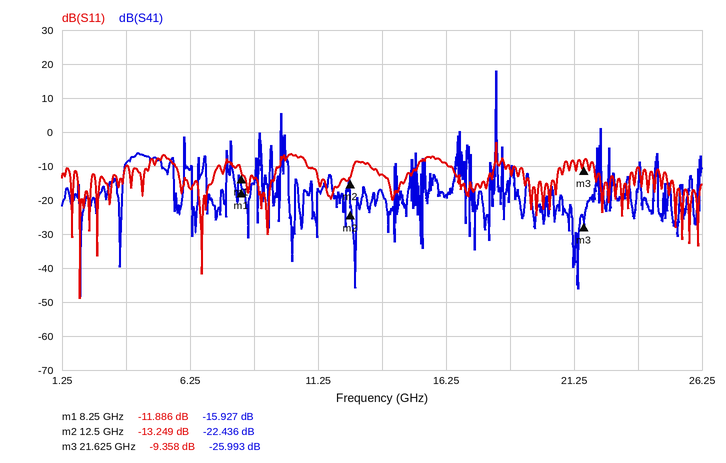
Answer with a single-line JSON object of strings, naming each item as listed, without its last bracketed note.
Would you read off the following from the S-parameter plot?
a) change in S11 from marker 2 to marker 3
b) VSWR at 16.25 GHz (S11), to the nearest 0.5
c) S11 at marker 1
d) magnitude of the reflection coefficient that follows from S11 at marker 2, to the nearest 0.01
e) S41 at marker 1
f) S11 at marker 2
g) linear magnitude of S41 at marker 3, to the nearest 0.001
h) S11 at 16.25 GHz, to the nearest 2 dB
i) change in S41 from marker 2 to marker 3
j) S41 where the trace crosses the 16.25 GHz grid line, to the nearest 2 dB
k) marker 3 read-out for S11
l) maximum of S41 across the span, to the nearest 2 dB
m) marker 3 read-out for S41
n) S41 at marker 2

{"change in S11 from marker 2 to marker 3": "3.891 dB", "VSWR at 16.25 GHz (S11), to the nearest 0.5": "2.0", "S11 at marker 1": "-11.886 dB", "magnitude of the reflection coefficient that follows from S11 at marker 2, to the nearest 0.01": "0.22", "S41 at marker 1": "-15.927 dB", "S11 at marker 2": "-13.249 dB", "linear magnitude of S41 at marker 3, to the nearest 0.001": "0.050", "S11 at 16.25 GHz, to the nearest 2 dB": "-10 dB", "change in S41 from marker 2 to marker 3": "-3.557 dB", "S41 where the trace crosses the 16.25 GHz grid line, to the nearest 2 dB": "-18 dB", "marker 3 read-out for S11": "-9.358 dB", "maximum of S41 across the span, to the nearest 2 dB": "18 dB", "marker 3 read-out for S41": "-25.993 dB", "S41 at marker 2": "-22.436 dB"}
